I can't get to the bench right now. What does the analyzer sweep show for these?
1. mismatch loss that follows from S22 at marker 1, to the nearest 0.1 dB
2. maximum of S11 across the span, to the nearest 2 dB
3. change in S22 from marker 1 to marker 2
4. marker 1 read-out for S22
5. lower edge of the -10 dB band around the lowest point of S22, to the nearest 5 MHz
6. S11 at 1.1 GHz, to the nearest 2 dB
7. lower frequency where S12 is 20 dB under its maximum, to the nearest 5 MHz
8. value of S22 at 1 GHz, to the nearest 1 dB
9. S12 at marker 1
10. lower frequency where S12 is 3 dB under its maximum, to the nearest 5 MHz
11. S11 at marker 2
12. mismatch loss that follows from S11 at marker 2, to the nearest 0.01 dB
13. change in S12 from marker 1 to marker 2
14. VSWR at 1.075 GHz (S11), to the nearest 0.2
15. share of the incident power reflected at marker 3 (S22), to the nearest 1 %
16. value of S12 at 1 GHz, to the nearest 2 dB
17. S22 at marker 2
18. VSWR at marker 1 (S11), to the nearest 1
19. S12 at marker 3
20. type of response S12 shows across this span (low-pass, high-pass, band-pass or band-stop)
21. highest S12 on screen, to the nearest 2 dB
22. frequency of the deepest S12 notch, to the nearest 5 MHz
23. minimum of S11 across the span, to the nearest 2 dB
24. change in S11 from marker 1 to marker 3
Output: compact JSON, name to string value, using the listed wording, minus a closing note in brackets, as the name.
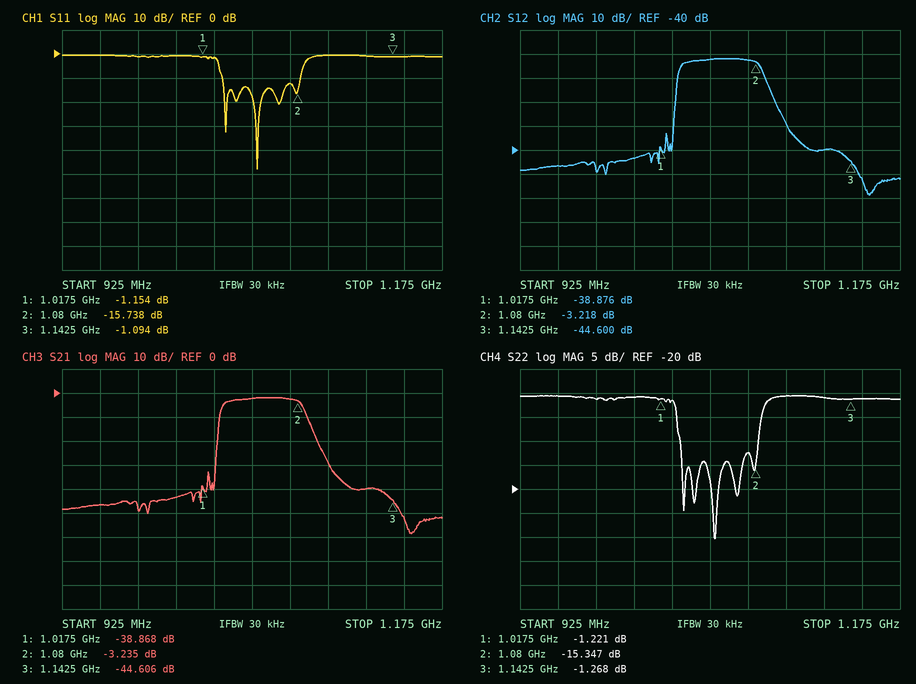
{"mismatch loss that follows from S22 at marker 1, to the nearest 0.1 dB": "6.1 dB", "maximum of S11 across the span, to the nearest 2 dB": "0 dB", "change in S22 from marker 1 to marker 2": "-14.126 dB", "marker 1 read-out for S22": "-1.221 dB", "lower edge of the -10 dB band around the lowest point of S22, to the nearest 5 MHz": "1.030 GHz", "S11 at 1.1 GHz, to the nearest 2 dB": "0 dB", "lower frequency where S12 is 20 dB under its maximum, to the nearest 5 MHz": "1.025 GHz", "value of S22 at 1 GHz, to the nearest 1 dB": "-1 dB", "S12 at marker 1": "-38.876 dB", "lower frequency where S12 is 3 dB under its maximum, to the nearest 5 MHz": "1.030 GHz", "S11 at marker 2": "-15.738 dB", "mismatch loss that follows from S11 at marker 2, to the nearest 0.01 dB": "0.12 dB", "change in S12 from marker 1 to marker 2": "35.658 dB", "VSWR at 1.075 GHz (S11), to the nearest 0.2": "1.6", "share of the incident power reflected at marker 3 (S22), to the nearest 1 %": "75 %", "value of S12 at 1 GHz, to the nearest 2 dB": "-44 dB", "S22 at marker 2": "-15.347 dB", "VSWR at marker 1 (S11), to the nearest 1": "15", "S12 at marker 3": "-44.600 dB", "type of response S12 shows across this span": "band-pass", "highest S12 on screen, to the nearest 2 dB": "-2 dB", "frequency of the deepest S12 notch, to the nearest 5 MHz": "1.155 GHz", "minimum of S11 across the span, to the nearest 2 dB": "-48 dB", "change in S11 from marker 1 to marker 3": "0.060 dB"}
